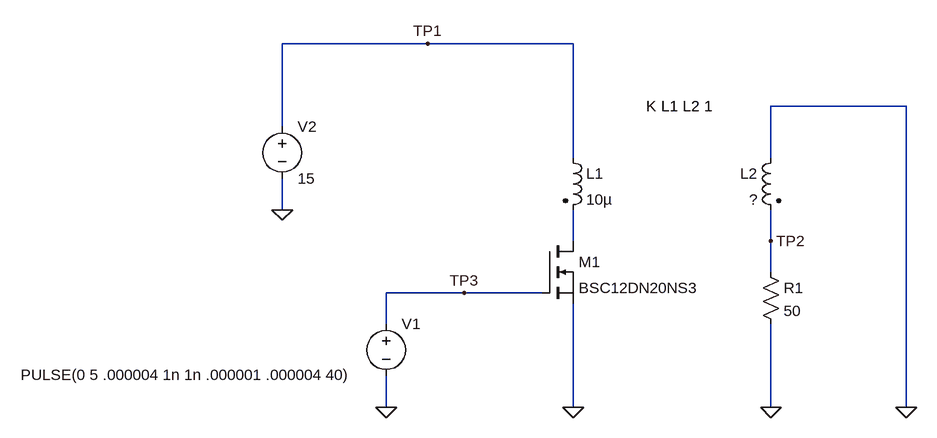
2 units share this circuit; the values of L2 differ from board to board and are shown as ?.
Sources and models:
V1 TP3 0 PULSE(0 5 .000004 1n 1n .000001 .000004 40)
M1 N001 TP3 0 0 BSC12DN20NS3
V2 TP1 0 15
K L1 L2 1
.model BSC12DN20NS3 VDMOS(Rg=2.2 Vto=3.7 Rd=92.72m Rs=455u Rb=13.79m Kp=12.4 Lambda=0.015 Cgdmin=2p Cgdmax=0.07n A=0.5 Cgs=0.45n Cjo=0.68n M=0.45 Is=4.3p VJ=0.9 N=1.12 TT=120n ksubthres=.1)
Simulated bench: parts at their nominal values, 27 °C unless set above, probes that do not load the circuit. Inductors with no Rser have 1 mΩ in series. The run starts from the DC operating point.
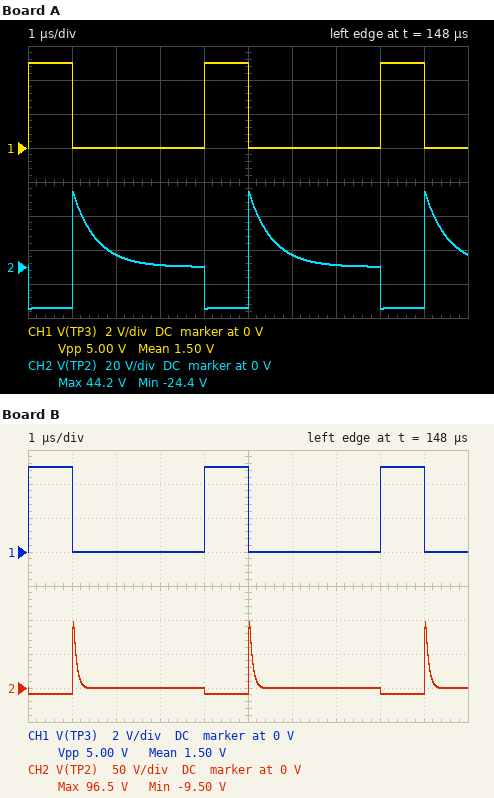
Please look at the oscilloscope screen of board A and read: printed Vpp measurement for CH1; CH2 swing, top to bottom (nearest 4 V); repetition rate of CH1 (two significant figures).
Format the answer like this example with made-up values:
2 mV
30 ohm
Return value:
5.00 V
68 V
250 kHz
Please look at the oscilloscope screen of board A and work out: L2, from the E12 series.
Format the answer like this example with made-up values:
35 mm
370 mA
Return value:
27 µH
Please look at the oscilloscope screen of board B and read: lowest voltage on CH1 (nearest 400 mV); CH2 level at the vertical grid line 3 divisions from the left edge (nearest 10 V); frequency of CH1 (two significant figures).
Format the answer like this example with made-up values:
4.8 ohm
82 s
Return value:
0 V
0 V
250 kHz
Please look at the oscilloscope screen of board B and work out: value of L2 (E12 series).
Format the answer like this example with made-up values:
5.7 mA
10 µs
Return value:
3.9 µH
